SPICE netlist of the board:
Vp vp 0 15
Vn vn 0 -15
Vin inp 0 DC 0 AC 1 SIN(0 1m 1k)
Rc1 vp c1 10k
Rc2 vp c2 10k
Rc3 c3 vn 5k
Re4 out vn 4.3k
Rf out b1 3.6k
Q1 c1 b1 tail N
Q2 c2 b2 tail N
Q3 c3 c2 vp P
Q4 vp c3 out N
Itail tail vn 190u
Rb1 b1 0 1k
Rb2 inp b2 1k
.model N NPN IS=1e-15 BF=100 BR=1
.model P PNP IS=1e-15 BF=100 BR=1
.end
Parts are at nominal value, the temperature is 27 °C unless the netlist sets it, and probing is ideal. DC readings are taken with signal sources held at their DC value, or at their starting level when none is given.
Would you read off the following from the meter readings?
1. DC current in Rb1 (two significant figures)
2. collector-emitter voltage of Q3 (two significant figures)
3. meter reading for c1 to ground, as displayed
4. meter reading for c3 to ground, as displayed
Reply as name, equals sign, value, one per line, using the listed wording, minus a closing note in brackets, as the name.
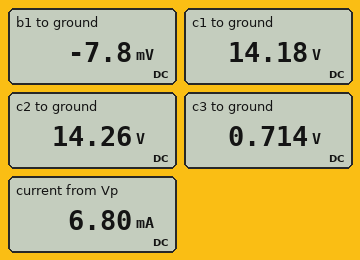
DC current in Rb1 = 7.8 µA
collector-emitter voltage of Q3 = -14 V
meter reading for c1 to ground, as displayed = 14.18 V
meter reading for c3 to ground, as displayed = 0.714 V
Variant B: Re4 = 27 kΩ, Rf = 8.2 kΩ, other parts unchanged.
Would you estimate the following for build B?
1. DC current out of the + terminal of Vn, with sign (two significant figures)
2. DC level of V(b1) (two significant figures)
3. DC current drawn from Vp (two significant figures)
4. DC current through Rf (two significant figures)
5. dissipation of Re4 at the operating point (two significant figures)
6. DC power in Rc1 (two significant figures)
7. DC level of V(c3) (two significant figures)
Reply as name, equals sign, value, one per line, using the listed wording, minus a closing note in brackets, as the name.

DC current out of the + terminal of Vn, with sign = -3.9 mA
DC level of V(b1) = -7.5 mV
DC current drawn from Vp = 3.9 mA
DC current through Rf = 6.7 µA
dissipation of Re4 at the operating point = 8.3 mW
DC power in Rc1 = 68 µW
DC level of V(c3) = 640 mV
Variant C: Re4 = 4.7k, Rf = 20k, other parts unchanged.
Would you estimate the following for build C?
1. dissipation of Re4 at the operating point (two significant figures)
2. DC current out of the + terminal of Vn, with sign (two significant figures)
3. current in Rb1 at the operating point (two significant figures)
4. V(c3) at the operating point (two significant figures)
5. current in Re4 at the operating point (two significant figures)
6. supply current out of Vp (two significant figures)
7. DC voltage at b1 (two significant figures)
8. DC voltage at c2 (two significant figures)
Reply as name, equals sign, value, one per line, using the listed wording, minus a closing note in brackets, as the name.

dissipation of Re4 at the operating point = 47 mW
DC current out of the + terminal of Vn, with sign = -6.5 mA
current in Rb1 at the operating point = 7.6 µA
V(c3) at the operating point = 600 mV
current in Re4 at the operating point = 3.2 mA
supply current out of Vp = 6.5 mA
DC voltage at b1 = -7.6 mV
DC voltage at c2 = 14 V
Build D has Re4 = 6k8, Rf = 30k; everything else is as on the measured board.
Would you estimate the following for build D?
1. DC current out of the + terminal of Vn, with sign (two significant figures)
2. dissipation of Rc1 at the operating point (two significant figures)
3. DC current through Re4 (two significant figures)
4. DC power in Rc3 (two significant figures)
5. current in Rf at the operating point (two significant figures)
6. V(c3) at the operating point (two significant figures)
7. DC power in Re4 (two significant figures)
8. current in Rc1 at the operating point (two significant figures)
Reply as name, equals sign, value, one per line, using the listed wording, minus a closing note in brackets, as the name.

DC current out of the + terminal of Vn, with sign = -5.5 mA
dissipation of Rc1 at the operating point = 68 µW
DC current through Re4 = 2.2 mA
DC power in Rc3 = 48 mW
current in Rf at the operating point = 6.7 µA
V(c3) at the operating point = 530 mV
DC power in Re4 = 32 mW
current in Rc1 at the operating point = 82 µA
